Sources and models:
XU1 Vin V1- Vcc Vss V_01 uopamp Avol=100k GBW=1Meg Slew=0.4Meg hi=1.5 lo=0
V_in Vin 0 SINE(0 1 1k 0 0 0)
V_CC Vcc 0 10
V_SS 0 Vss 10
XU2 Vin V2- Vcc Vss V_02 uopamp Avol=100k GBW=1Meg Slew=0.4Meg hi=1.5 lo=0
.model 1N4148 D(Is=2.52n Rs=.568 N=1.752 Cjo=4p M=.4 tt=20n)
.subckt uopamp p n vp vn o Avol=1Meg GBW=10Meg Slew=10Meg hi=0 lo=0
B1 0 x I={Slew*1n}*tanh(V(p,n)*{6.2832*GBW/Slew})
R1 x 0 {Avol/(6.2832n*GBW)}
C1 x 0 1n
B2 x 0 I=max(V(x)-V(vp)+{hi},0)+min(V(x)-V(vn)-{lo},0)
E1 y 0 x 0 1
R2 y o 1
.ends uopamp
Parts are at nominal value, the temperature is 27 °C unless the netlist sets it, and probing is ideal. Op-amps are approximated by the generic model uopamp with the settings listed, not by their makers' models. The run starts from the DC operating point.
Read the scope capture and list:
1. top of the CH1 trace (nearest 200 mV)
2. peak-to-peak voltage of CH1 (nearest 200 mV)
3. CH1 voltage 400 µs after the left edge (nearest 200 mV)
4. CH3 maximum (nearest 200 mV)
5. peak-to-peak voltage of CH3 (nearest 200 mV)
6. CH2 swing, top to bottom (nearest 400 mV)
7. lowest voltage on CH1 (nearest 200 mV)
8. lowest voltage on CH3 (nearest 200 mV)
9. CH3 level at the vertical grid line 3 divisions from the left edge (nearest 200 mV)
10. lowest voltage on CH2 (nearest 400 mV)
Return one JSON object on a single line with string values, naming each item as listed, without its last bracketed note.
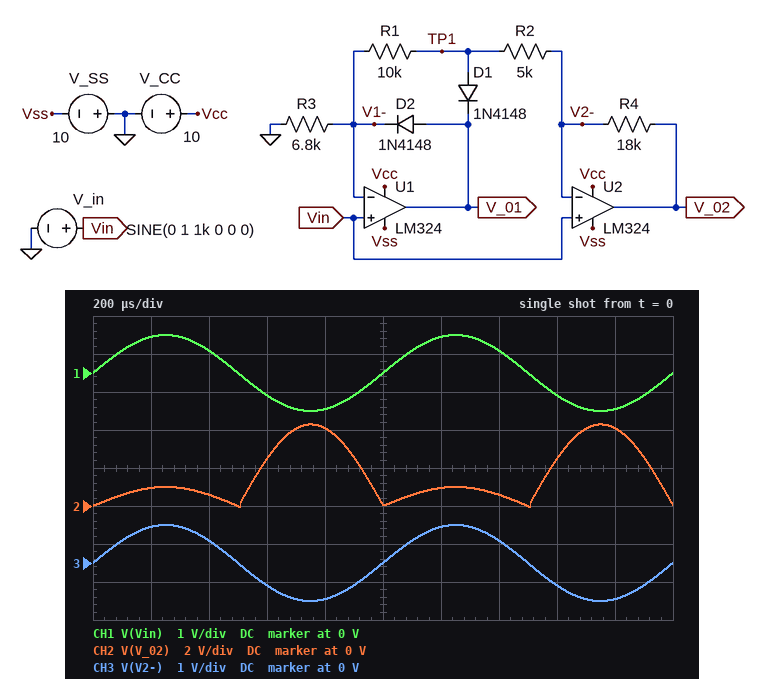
{"top of the CH1 trace": "1.0 V", "peak-to-peak voltage of CH1": "2.0 V", "CH1 voltage 400 µs after the left edge": "600 mV", "CH3 maximum": "1.0 V", "peak-to-peak voltage of CH3": "2.0 V", "CH2 swing, top to bottom": "4.4 V", "lowest voltage on CH1": "-1.0 V", "lowest voltage on CH3": "-1.0 V", "CH3 level at the vertical grid line 3 divisions from the left edge": "-600 mV", "lowest voltage on CH2": "0 V"}
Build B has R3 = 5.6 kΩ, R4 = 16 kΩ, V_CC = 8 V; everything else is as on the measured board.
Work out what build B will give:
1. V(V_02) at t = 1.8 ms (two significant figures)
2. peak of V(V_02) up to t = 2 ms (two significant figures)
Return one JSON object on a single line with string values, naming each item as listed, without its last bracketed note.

{"V(V_02) at t = 1.8 ms": "4.5 V", "peak of V(V_02) up to t = 2 ms": "4.7 V"}
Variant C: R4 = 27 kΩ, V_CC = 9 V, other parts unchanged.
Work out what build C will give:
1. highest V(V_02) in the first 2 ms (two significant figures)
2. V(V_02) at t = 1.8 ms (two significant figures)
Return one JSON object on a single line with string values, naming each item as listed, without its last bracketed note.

{"highest V(V_02) in the first 2 ms": "6.9 V", "V(V_02) at t = 1.8 ms": "6.6 V"}
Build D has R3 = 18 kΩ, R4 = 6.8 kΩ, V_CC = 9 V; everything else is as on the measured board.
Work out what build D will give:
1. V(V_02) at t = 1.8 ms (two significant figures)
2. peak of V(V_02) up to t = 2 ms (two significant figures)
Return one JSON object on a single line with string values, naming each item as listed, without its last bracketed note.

{"V(V_02) at t = 1.8 ms": "-230 mV", "peak of V(V_02) up to t = 2 ms": "1.0 V"}
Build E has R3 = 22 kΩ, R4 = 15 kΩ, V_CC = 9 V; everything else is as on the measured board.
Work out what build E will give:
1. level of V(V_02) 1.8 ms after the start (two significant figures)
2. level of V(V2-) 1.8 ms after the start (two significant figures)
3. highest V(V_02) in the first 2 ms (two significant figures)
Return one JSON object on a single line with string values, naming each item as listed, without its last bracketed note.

{"level of V(V_02) 1.8 ms after the start": "350 mV", "level of V(V2-) 1.8 ms after the start": "-950 mV", "highest V(V_02) in the first 2 ms": "1.0 V"}
